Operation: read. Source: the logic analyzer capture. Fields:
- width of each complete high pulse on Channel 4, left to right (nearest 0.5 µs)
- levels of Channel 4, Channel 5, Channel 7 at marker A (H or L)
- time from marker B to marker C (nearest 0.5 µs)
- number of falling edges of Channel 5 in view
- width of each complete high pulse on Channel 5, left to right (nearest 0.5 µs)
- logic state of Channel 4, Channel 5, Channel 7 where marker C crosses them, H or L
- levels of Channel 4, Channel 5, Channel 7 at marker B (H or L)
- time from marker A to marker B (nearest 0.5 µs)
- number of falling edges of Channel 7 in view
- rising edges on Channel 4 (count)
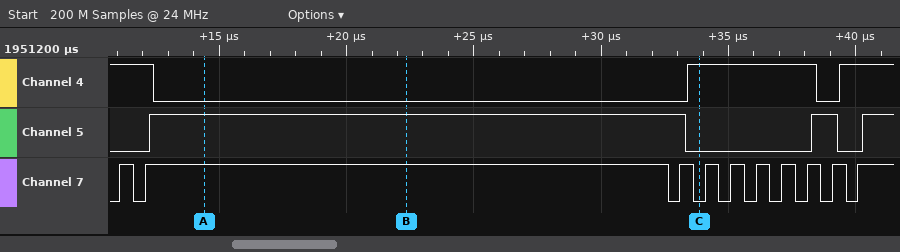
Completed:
5 µs
Channel 4=L, Channel 5=H, Channel 7=H
11.5 µs
2
21 µs, 1 µs
Channel 4=H, Channel 5=L, Channel 7=L
Channel 4=L, Channel 5=H, Channel 7=H
8 µs
9
2
